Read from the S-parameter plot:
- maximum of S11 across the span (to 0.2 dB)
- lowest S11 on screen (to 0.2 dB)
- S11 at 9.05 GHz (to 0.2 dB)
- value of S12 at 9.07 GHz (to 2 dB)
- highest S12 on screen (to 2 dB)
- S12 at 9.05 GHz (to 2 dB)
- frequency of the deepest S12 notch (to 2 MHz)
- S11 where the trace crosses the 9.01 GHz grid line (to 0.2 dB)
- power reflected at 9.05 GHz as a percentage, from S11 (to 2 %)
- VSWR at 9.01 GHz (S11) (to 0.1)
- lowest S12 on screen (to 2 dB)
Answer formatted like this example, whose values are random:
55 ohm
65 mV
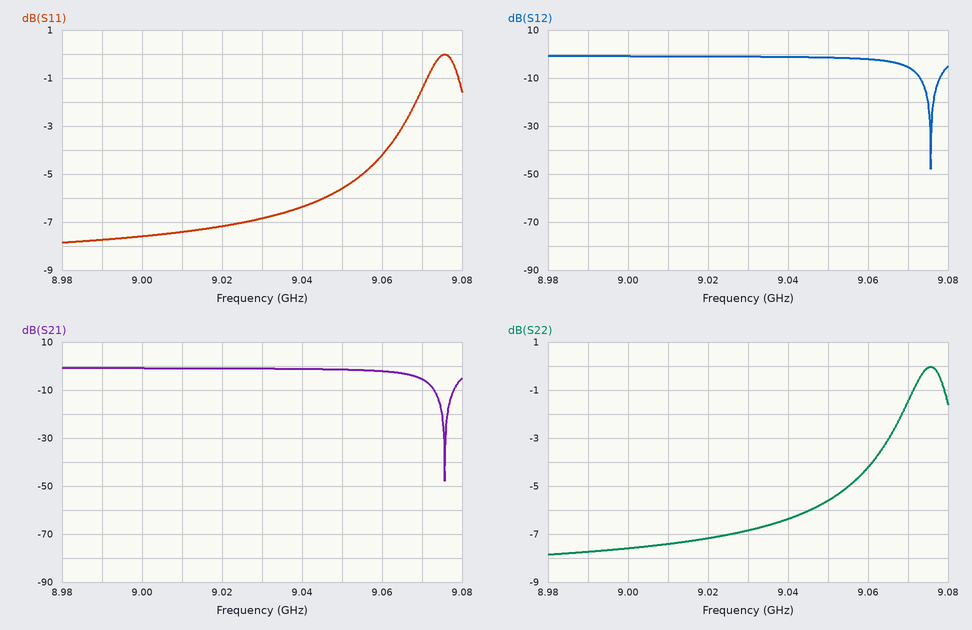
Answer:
0.0 dB
-7.8 dB
-5.6 dB
-6 dB
0 dB
-2 dB
9.076 GHz
-7.4 dB
28 %
2.5
-48 dB
